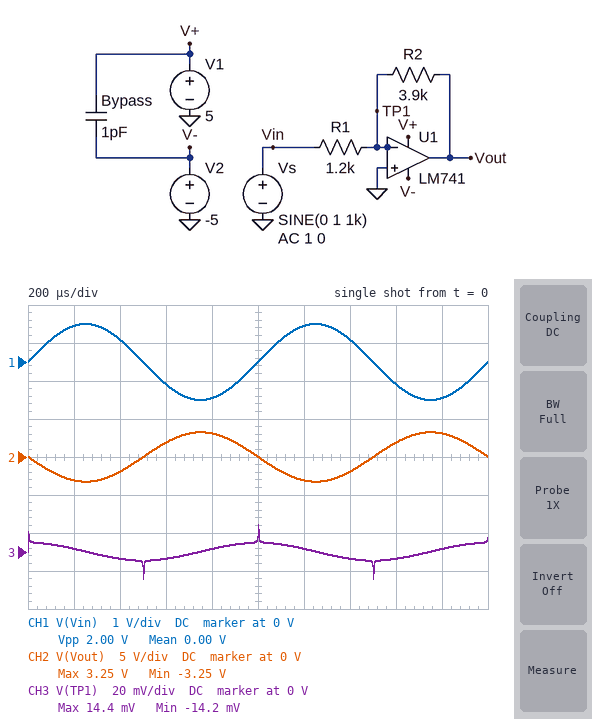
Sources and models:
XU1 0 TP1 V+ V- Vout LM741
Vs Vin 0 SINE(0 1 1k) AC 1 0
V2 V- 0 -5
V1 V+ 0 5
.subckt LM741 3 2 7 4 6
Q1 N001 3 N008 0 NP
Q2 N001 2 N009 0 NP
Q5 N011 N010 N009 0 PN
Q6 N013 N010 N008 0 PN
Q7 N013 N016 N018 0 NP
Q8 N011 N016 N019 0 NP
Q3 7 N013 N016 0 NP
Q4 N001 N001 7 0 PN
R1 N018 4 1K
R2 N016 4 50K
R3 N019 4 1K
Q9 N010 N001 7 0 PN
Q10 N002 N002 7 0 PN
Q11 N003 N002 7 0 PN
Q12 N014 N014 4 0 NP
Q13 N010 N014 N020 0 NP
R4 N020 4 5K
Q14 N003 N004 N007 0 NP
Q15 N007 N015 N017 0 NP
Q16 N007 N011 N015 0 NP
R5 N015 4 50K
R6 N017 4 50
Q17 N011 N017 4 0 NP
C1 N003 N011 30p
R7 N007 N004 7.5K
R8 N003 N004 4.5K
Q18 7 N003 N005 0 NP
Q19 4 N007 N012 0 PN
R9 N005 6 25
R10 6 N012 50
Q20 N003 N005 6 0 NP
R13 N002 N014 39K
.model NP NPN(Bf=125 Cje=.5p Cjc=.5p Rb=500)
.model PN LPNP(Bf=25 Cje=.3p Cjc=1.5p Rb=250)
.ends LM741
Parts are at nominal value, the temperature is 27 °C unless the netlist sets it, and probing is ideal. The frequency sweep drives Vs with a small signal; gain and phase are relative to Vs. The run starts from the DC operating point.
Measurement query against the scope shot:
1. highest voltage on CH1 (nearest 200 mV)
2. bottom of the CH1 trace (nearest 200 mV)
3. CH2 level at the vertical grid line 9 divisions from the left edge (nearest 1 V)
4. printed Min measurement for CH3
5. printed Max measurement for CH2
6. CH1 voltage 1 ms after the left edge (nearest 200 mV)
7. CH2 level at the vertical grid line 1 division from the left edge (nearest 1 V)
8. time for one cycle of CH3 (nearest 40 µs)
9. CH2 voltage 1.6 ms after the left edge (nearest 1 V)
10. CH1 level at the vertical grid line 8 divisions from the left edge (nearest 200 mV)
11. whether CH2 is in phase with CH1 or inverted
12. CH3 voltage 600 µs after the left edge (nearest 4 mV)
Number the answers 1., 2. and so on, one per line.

1. 1.0 V
2. -1.0 V
3. 3 V
4. -14.2 mV
5. 3.25 V
6. 0 V
7. -3 V
8. 1.00 ms
9. 2 V
10. -600 mV
11. inverted
12. -4 mV
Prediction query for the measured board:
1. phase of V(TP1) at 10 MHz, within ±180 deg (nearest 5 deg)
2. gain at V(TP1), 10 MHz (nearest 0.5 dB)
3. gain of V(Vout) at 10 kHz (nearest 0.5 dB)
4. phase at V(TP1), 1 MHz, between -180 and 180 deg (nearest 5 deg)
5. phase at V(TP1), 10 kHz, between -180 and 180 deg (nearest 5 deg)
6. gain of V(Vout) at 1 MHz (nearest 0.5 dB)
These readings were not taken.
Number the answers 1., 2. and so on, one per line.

1. -5 deg
2. -0.5 dB
3. 9.5 dB
4. 0 deg
5. 70 deg
6. -1.5 dB
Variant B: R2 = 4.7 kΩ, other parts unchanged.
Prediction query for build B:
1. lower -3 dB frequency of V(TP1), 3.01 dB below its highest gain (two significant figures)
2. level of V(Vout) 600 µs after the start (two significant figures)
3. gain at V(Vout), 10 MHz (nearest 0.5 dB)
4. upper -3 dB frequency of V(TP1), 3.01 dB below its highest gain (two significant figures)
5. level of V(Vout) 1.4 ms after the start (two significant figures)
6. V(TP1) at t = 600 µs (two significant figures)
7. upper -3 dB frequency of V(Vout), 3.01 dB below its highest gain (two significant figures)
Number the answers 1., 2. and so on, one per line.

1. 26 kHz
2. 2.3 V
3. -3.0 dB
4. 130 MHz
5. -2.3 V
6. -4.3 mV
7. 27 kHz
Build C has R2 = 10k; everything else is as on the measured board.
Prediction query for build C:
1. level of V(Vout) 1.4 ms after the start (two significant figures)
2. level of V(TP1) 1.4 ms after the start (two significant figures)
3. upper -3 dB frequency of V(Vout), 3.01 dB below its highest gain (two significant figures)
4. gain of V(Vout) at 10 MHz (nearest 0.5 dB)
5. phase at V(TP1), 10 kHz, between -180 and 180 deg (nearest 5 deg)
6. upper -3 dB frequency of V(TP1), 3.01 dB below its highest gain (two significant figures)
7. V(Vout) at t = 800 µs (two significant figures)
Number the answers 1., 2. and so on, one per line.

1. -3.5 V
2. 150 mV
3. 23 kHz
4. -5.5 dB
5. 65 deg
6. 170 MHz
7. 4.2 V
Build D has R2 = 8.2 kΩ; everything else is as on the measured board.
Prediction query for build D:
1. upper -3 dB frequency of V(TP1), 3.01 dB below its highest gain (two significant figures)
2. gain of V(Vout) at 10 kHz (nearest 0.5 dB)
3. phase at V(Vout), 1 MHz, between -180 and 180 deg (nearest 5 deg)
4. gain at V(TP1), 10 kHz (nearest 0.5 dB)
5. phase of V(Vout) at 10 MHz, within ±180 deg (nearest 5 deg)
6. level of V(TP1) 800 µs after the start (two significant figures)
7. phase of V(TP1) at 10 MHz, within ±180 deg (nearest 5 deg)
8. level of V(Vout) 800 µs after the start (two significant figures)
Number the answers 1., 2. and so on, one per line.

1. 160 MHz
2. 16.0 dB
3. 10 deg
4. -8.5 dB
5. -35 deg
6. -290 mV
7. -5 deg
8. 4.2 V
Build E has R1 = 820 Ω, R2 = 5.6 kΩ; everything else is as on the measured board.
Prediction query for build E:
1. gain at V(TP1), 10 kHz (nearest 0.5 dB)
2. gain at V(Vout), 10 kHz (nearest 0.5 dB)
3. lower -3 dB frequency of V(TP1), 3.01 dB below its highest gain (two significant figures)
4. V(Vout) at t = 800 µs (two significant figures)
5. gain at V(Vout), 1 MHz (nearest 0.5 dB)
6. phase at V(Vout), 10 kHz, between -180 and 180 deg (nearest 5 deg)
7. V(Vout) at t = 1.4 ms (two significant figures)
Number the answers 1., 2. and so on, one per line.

1. -6.5 dB
2. 15.5 dB
3. 18 kHz
4. 4.2 V
5. -2.0 dB
6. 145 deg
7. -3.4 V
